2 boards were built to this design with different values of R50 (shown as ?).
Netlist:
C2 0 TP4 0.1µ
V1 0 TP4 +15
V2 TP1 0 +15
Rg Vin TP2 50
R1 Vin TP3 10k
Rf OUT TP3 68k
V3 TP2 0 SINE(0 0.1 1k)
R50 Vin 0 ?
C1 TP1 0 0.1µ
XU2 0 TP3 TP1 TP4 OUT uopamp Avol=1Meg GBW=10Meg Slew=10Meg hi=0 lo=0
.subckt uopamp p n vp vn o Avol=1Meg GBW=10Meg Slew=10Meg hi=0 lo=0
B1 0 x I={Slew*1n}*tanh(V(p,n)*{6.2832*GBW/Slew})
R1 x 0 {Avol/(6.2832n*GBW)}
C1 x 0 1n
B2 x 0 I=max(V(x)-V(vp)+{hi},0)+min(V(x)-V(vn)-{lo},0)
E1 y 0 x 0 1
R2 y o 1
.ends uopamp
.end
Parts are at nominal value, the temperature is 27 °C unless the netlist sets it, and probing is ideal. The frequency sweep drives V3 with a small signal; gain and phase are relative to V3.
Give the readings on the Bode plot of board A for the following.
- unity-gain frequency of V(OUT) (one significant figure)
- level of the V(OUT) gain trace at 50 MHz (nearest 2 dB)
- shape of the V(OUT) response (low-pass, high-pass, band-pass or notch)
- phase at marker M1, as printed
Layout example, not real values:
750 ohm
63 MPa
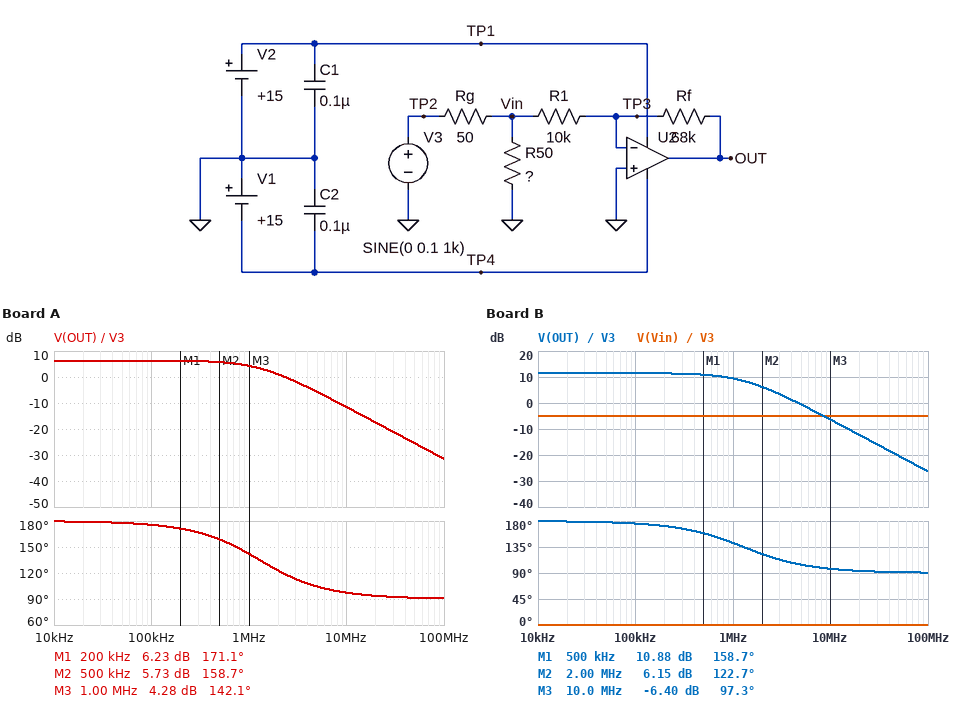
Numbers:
2 MHz
-26 dB
low-pass
171.1 deg
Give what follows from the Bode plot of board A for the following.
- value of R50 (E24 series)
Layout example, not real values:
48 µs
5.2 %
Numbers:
22 Ω
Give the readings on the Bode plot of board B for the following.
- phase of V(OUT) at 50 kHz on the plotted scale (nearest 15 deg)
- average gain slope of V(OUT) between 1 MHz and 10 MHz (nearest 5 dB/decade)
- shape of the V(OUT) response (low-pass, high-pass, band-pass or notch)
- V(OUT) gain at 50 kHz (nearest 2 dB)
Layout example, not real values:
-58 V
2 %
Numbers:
180 deg
-15 dB/decade
low-pass
12 dB
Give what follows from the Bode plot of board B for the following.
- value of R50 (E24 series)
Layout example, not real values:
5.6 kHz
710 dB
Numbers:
62 Ω
